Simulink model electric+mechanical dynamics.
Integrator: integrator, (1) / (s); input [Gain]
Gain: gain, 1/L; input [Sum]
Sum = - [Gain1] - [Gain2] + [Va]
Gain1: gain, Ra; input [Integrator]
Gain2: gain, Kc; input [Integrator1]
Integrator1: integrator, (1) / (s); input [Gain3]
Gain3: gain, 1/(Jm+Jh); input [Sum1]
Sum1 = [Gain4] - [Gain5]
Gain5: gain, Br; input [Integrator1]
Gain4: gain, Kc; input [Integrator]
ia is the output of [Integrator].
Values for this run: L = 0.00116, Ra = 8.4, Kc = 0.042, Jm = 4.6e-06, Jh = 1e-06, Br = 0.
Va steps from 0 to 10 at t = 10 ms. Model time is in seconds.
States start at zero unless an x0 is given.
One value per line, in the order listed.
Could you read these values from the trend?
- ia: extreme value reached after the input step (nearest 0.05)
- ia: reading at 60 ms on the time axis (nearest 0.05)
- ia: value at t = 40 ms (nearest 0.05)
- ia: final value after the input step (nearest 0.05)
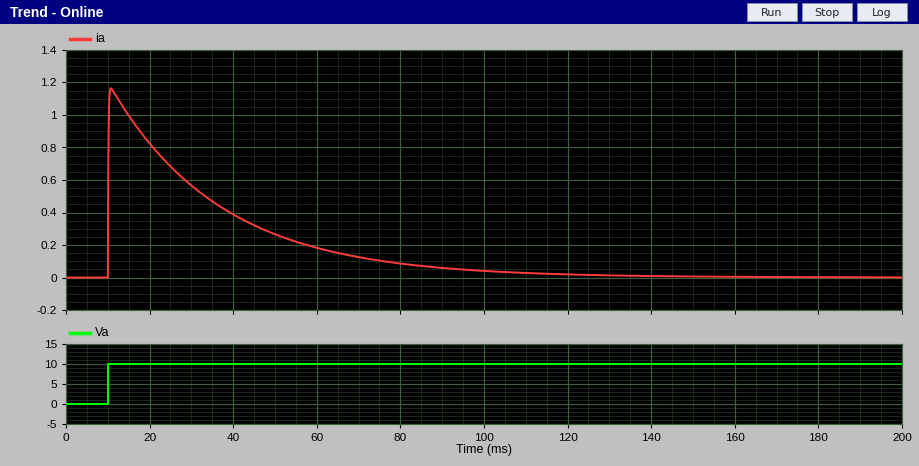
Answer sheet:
1.15
0.20
0.40
0.00
